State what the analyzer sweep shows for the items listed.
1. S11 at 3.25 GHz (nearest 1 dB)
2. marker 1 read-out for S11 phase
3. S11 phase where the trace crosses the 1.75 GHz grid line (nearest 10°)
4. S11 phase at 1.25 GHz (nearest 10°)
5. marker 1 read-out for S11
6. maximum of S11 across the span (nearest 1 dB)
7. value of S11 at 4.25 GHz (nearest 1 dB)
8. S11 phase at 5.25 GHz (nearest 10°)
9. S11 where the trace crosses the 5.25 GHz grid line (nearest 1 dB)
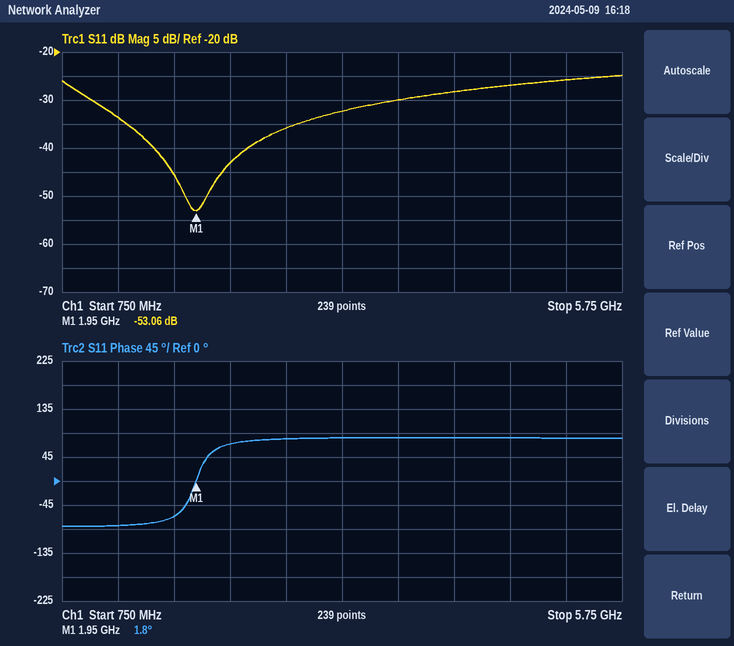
-32 dB
1.8°
-70°
-80°
-53.06 dB
-25 dB
-28 dB
80°
-26 dB
